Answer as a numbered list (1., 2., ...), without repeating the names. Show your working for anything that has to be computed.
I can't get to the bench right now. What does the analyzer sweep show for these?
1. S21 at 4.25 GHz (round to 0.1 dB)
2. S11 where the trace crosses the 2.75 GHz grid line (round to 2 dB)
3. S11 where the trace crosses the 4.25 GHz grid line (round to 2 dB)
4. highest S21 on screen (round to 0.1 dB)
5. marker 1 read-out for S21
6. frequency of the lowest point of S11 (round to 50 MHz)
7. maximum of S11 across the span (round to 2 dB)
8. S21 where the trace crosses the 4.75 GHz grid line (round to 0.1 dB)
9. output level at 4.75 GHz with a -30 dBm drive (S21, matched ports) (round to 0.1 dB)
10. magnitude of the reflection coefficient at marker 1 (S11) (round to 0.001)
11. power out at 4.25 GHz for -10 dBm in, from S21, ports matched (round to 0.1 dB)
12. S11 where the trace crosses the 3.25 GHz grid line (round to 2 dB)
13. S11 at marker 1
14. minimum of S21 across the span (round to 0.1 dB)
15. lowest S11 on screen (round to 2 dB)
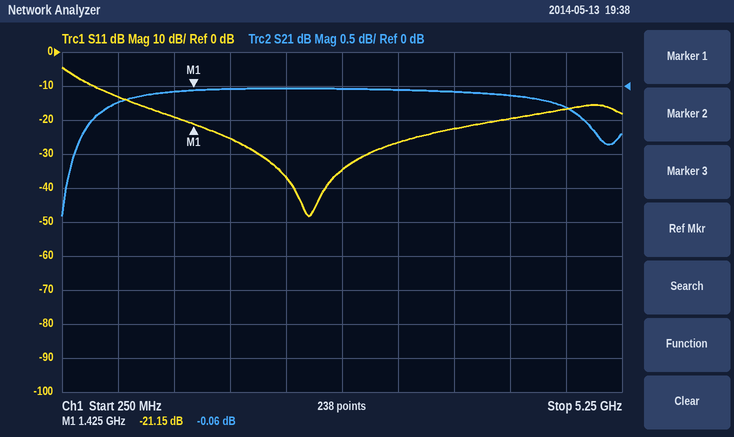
1. -0.1 dB
2. -34 dB
3. -20 dB
4. 0.0 dB
5. -0.06 dB
6. 2.45 GHz
7. -4 dB
8. -0.3 dB
9. -30 dBm + (-0.3 dB) = -30.3 dBm
10. 10^(-21.15/20) ≈ 0.088
11. -10 dBm + (-0.1 dB) = -10.1 dBm
12. -26 dB
13. -21.15 dB
14. -1.9 dB
15. -48 dB
